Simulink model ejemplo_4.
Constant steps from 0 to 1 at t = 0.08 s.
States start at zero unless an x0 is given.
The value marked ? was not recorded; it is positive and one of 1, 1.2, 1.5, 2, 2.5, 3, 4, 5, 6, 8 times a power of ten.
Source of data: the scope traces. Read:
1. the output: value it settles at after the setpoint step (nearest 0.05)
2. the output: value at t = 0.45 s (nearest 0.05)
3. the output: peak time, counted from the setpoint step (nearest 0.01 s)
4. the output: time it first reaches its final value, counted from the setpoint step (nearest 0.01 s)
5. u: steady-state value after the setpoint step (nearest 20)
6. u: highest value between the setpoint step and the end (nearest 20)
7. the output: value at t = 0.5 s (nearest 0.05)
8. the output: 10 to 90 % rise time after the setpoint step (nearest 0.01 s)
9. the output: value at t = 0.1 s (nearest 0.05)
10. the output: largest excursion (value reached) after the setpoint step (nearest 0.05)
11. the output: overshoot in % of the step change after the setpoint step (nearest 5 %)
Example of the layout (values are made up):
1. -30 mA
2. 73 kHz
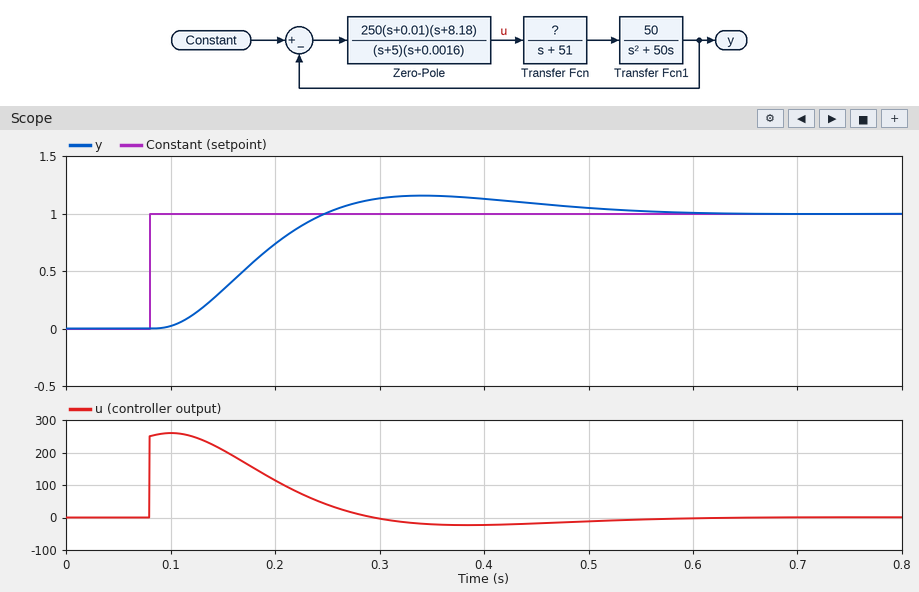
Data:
1. 1.00
2. 1.10
3. 0.26 s
4. 0.17 s
5. 0
6. 260
7. 1.05
8. 0.11 s
9. 0.00
10. 1.15
11. 15 %
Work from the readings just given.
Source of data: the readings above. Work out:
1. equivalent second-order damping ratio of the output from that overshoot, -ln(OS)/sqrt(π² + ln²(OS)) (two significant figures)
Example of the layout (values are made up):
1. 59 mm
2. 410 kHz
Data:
1. 0.52
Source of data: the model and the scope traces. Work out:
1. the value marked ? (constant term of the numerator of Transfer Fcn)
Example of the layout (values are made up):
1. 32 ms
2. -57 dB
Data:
1. 2
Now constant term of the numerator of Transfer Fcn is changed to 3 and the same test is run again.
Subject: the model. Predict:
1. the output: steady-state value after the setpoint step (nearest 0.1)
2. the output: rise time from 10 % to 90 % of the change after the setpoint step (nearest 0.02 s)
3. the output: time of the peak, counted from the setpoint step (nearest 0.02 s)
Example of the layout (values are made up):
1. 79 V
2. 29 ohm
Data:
1. 1.0
2. 0.08 s
3. 0.18 s
